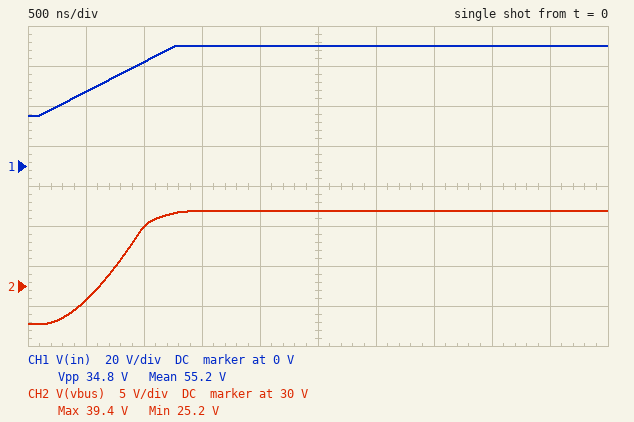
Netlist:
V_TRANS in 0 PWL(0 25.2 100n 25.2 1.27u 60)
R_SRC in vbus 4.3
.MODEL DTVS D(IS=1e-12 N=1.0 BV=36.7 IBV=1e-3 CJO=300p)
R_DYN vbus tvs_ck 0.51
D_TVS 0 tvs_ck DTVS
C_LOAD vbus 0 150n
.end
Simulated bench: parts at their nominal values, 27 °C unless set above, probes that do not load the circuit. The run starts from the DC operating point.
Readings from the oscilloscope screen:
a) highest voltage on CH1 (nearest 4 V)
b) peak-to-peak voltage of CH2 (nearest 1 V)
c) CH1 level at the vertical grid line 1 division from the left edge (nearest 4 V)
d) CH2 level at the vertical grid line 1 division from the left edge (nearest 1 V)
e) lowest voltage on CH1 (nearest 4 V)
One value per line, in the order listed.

60 V
14 V
36 V
28 V
24 V
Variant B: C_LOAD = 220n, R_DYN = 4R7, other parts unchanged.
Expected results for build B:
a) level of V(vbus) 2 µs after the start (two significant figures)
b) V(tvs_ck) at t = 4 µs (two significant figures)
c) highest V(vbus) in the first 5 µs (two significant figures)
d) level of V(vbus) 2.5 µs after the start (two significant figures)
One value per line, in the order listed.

47 V
37 V
49 V
48 V
